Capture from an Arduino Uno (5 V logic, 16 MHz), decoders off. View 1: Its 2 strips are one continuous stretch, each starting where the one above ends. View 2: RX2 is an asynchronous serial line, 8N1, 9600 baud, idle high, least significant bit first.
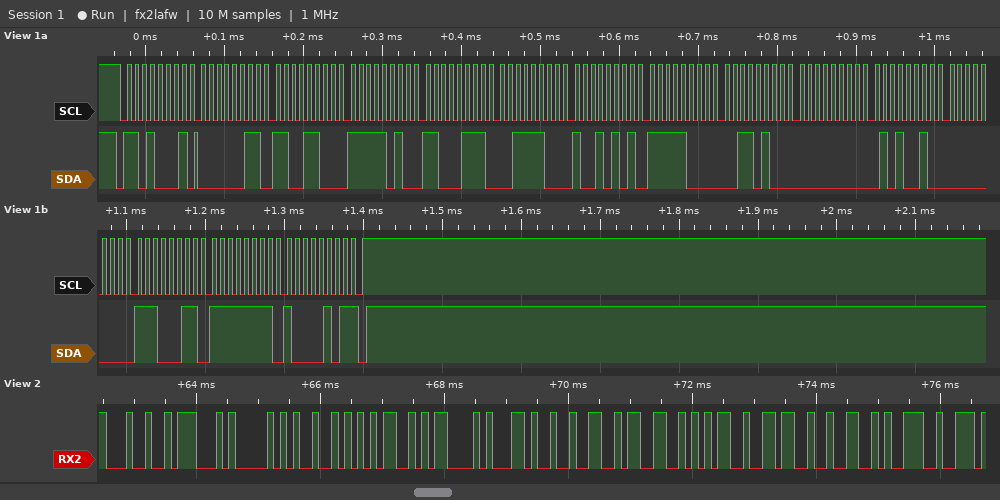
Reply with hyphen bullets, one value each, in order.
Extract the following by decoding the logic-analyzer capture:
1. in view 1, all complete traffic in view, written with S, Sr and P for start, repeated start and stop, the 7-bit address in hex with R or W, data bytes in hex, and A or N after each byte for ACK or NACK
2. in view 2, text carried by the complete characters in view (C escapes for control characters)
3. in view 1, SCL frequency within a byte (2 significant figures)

- S 68R A 03 A CC A FA A C7 A 3C A 95 A F8 A 34 A 00 A 52 A 00 A E3 A FF A 85 N P
- "$GPRMC,235629"
- 100 kHz
